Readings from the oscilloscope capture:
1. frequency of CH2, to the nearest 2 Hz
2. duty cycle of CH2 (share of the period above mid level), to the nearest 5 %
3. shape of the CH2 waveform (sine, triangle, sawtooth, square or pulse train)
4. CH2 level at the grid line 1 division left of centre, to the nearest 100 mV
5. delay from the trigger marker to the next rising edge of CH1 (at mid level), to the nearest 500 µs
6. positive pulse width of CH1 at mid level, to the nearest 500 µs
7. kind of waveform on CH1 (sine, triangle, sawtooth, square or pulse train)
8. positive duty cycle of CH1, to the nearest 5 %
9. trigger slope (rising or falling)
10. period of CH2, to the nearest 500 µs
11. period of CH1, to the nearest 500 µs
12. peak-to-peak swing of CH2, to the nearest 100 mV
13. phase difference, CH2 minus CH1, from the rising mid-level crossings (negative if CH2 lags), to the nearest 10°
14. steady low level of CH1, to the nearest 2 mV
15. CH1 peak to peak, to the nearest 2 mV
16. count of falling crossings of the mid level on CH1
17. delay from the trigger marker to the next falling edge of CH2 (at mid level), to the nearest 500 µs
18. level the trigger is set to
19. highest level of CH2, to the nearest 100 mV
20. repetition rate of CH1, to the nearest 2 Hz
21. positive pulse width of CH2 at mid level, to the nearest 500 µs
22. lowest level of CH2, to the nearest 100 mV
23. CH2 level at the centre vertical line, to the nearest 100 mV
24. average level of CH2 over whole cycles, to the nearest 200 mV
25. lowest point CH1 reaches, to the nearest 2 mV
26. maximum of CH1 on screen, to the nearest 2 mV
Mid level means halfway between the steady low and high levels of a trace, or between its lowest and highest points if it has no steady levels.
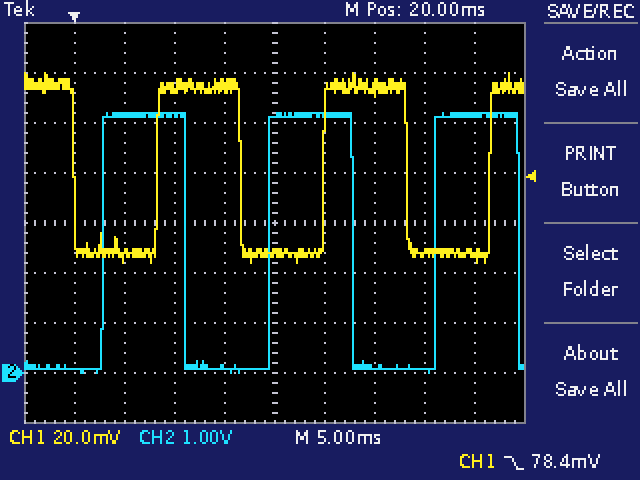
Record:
60 Hz
50 %
square
100 mV
8.5 ms
8.5 ms
square
50 %
falling
16.5 ms
16.5 ms
5.2 V
+120°
48 mV
76 mV
3
11.0 ms
78.4 mV
5.2 V
60 Hz
8.5 ms
0.0 V
5.2 V
2.6 V
44 mV
120 mV
